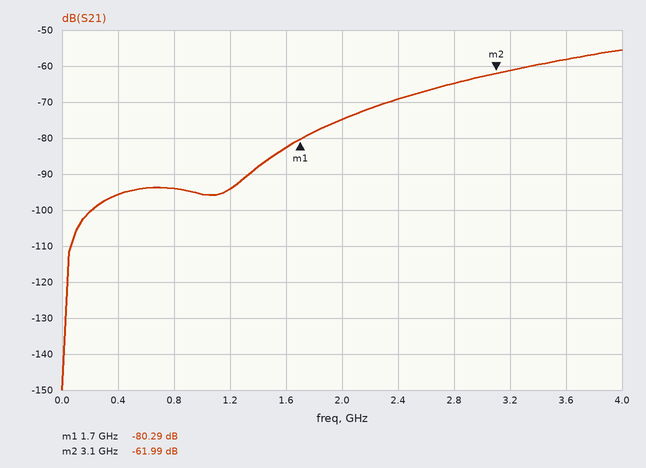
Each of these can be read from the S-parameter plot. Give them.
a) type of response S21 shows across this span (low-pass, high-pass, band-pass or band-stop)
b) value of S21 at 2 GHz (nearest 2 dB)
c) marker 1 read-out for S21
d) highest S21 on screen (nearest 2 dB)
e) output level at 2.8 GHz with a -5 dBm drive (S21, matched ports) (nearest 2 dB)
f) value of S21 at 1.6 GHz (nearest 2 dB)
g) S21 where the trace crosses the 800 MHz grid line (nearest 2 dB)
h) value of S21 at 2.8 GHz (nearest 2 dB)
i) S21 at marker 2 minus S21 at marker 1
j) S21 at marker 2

high-pass
-74 dB
-80.29 dB
-56 dB
-70 dBm
-82 dB
-94 dB
-64 dB
18.30 dB
-61.99 dB
